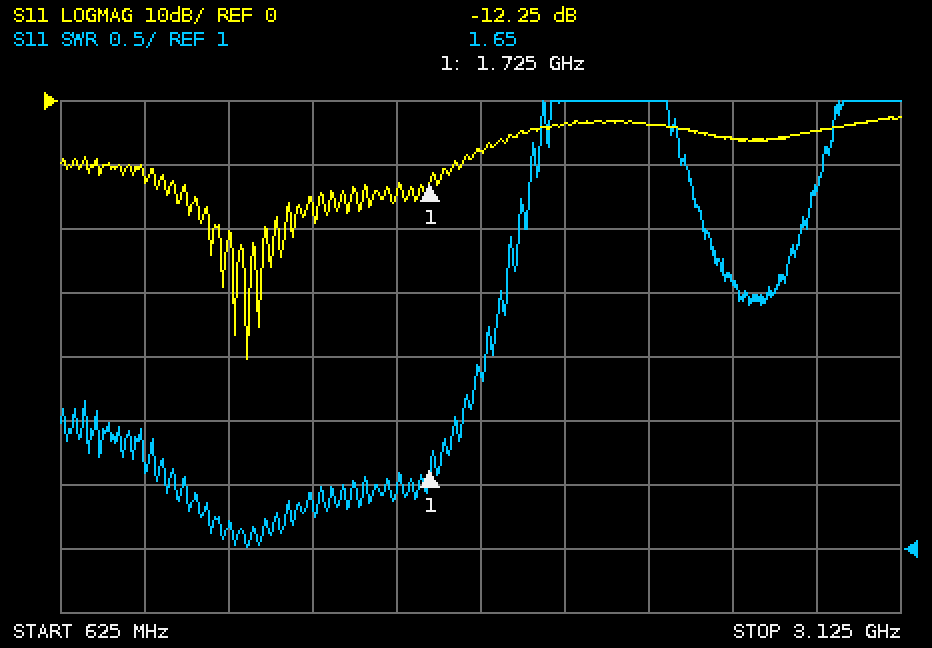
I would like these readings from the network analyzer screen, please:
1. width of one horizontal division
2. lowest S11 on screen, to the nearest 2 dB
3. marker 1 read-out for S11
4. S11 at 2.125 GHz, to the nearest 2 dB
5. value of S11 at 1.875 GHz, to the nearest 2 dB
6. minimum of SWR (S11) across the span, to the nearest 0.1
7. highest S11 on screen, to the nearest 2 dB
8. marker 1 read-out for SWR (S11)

250 MHz
-40 dB
-12.25 dB
-4 dB
-8 dB
1.0
-2 dB
1.65
